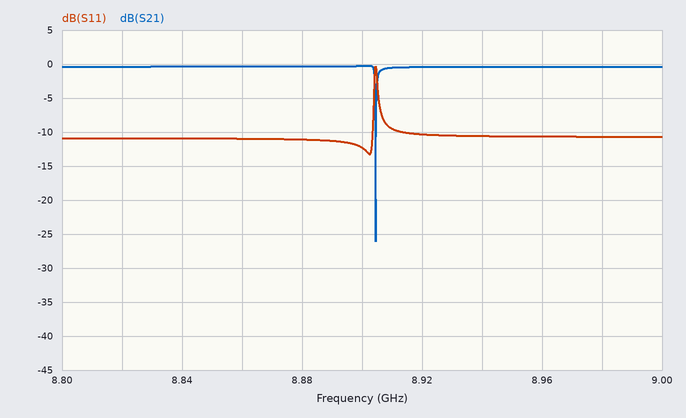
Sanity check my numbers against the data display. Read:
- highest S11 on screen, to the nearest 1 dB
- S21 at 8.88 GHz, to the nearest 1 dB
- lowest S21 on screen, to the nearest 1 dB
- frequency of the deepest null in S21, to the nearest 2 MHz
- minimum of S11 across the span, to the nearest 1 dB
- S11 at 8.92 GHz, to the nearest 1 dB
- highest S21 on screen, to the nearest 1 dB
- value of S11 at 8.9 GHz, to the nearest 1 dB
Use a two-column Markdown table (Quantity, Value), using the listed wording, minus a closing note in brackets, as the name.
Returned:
| Quantity | Value |
|---|---|
| highest S11 on screen, to the nearest 1 dB | 0 dB |
| S21 at 8.88 GHz, to the nearest 1 dB | 0 dB |
| lowest S21 on screen, to the nearest 1 dB | -26 dB |
| frequency of the deepest null in S21, to the nearest 2 MHz | 8.904 GHz |
| minimum of S11 across the span, to the nearest 1 dB | -13 dB |
| S11 at 8.92 GHz, to the nearest 1 dB | -10 dB |
| highest S21 on screen, to the nearest 1 dB | 0 dB |
| value of S11 at 8.9 GHz, to the nearest 1 dB | -12 dB |
